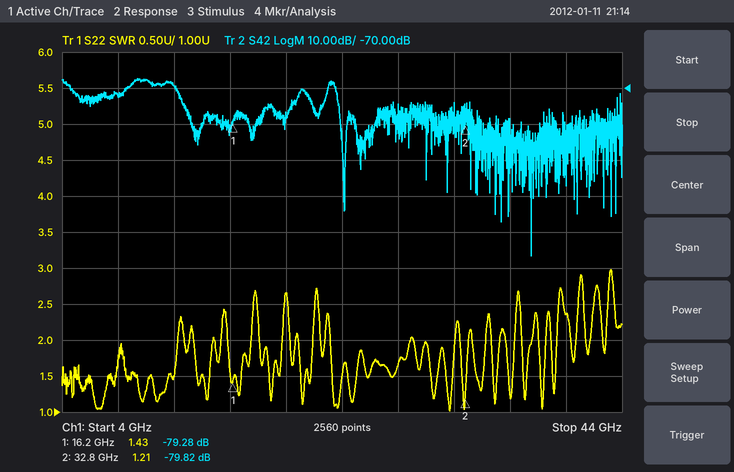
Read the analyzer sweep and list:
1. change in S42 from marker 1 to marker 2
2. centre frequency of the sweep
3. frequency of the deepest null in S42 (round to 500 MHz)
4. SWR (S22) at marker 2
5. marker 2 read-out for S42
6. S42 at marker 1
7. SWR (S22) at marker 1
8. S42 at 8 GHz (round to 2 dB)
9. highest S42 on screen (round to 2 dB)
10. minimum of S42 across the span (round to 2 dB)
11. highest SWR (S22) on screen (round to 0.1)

-0.54 dB
24 GHz
37.5 GHz
1.21
-79.82 dB
-79.28 dB
1.43
-72 dB
-68 dB
-116 dB
3.0
